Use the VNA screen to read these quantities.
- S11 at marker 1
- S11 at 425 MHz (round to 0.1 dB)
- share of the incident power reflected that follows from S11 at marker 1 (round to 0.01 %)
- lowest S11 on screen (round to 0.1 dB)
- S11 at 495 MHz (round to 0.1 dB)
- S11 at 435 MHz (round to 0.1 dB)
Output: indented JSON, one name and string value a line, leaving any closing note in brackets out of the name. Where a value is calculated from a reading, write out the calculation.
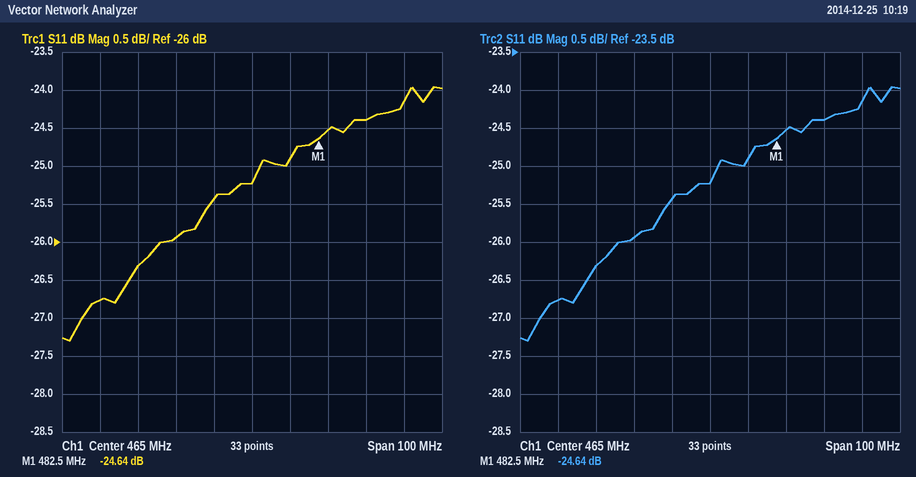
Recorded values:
{
  "S11 at marker 1": "-24.64 dB",
  "S11 at 425 MHz": "-26.8 dB",
  "share of the incident power reflected that follows from S11 at marker 1": "10^(-24.64/10) ≈ 0.34 %",
  "lowest S11 on screen": "-27.3 dB",
  "S11 at 495 MHz": "-24.4 dB",
  "S11 at 435 MHz": "-26.3 dB"
}
